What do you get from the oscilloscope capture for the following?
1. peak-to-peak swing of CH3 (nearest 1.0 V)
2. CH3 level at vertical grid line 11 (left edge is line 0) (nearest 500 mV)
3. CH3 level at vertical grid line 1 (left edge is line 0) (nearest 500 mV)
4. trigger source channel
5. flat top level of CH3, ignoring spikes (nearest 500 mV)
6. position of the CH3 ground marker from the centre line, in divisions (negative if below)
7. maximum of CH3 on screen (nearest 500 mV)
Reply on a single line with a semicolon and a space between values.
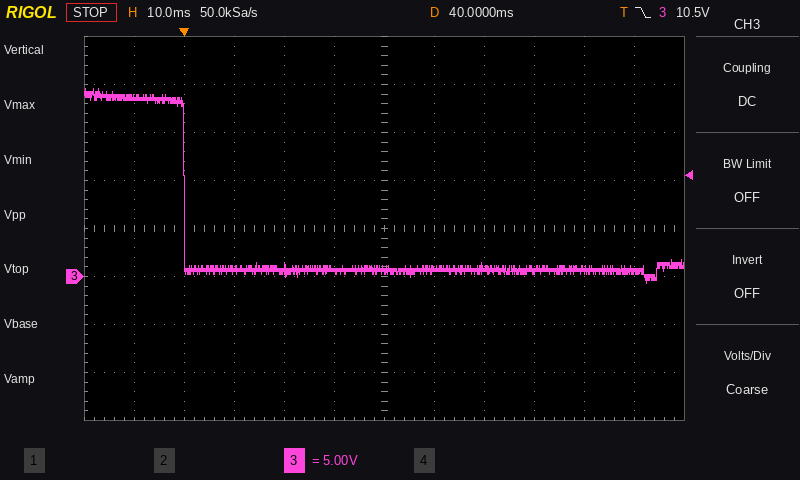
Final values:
20.0 V; 500 mV; 18.5 V; CH3; 18.5 V; -1.0 div; 19.5 V
